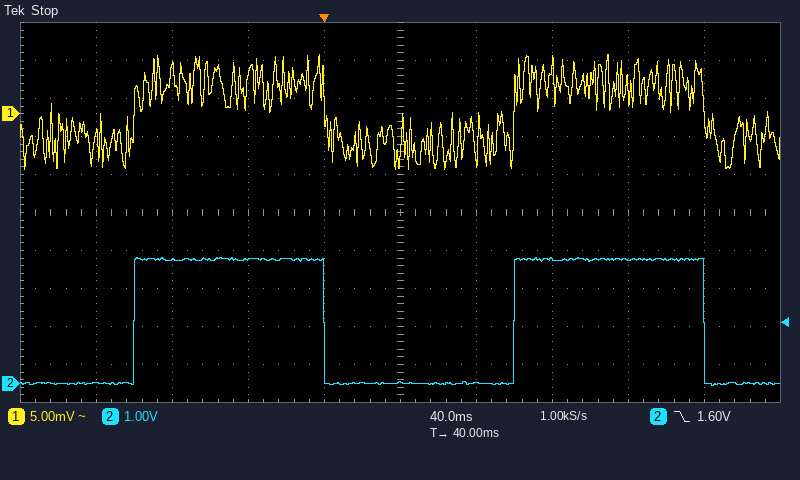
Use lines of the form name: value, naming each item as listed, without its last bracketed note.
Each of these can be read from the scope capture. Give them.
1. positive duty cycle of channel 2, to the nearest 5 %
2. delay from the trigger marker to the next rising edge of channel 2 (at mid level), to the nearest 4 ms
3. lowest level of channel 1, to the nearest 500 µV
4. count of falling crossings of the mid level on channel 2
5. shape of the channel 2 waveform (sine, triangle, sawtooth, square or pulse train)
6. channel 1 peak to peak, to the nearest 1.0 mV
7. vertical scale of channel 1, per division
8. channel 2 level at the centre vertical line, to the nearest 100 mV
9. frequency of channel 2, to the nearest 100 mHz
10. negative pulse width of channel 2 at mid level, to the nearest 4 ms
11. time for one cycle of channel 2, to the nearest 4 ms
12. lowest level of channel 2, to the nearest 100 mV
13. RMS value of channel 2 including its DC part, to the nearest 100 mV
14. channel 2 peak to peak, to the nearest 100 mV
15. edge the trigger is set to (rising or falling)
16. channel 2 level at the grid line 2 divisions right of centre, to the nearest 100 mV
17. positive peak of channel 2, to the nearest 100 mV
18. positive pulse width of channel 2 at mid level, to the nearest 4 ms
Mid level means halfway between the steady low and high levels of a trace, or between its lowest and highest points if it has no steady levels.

positive duty cycle of channel 2, to the nearest 5 %: 50 %
delay from the trigger marker to the next rising edge of channel 2 (at mid level), to the nearest 4 ms: 100 ms
lowest level of channel 1, to the nearest 500 µV: -7.5 mV
count of falling crossings of the mid level on channel 2: 2
shape of the channel 2 waveform: square
channel 1 peak to peak, to the nearest 1.0 mV: 15.0 mV
vertical scale of channel 1, per division: 5 mV
channel 2 level at the centre vertical line, to the nearest 100 mV: 0.0 V
frequency of channel 2, to the nearest 100 mHz: 5.0 Hz
negative pulse width of channel 2 at mid level, to the nearest 4 ms: 100 ms
time for one cycle of channel 2, to the nearest 4 ms: 200 ms
lowest level of channel 2, to the nearest 100 mV: -100 mV
RMS value of channel 2 including its DC part, to the nearest 100 mV: 2.3 V
channel 2 peak to peak, to the nearest 100 mV: 3.4 V
edge the trigger is set to: falling
channel 2 level at the grid line 2 divisions right of centre, to the nearest 100 mV: 3.3 V
positive peak of channel 2, to the nearest 100 mV: 3.3 V
positive pulse width of channel 2 at mid level, to the nearest 4 ms: 100 ms
